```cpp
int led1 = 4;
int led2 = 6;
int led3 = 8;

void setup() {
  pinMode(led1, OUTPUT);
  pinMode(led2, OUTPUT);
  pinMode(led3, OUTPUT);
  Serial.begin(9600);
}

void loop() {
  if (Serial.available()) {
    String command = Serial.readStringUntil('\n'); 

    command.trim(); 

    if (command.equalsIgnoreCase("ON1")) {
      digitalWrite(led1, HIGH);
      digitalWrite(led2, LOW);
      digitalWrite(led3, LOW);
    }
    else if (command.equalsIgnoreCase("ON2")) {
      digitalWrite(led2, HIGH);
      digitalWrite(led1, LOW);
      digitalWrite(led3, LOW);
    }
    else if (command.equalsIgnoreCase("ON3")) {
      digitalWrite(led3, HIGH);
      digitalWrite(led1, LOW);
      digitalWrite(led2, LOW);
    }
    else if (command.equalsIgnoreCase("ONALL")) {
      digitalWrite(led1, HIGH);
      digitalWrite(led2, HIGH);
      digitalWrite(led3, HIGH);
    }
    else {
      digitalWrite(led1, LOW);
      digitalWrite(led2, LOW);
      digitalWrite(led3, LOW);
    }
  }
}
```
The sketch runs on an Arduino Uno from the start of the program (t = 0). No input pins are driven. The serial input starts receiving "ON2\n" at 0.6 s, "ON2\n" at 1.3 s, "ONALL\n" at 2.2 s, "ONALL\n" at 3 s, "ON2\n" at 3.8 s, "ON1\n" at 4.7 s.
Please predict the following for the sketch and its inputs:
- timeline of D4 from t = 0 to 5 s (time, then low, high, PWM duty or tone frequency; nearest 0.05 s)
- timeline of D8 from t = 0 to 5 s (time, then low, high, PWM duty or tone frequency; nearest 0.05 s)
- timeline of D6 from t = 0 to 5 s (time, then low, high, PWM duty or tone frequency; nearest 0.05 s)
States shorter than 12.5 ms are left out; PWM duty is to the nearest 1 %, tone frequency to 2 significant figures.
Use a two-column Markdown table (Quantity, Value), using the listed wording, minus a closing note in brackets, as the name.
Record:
| Quantity | Value |
|---|---|
| timeline of D4 from t = 0 to 5 s | 0 s low; 2.2 s high; 3.8 s low; 4.7 s high |
| timeline of D8 from t = 0 to 5 s | 0 s low; 2.2 s high; 3.8 s low |
| timeline of D6 from t = 0 to 5 s | 0 s low; 0.6 s high; 4.7 s low |
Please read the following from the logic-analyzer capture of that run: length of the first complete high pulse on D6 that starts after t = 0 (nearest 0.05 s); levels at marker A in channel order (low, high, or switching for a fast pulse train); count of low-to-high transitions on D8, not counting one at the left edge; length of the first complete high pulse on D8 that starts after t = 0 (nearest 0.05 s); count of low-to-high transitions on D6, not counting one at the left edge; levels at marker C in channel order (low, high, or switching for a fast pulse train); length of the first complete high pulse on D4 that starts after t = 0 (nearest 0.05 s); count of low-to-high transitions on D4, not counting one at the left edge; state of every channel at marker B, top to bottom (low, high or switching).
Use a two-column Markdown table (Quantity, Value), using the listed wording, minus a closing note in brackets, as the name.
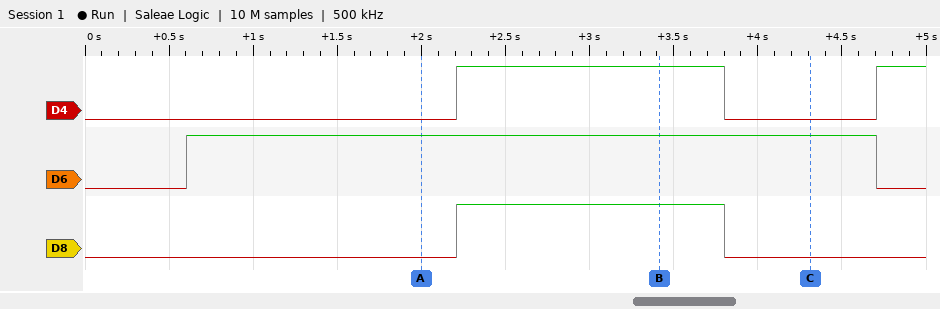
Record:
| Quantity | Value |
|---|---|
| length of the first complete high pulse on D6 that starts after t = 0 | 4.10 s |
| levels at marker A in channel order | D4 low, D6 high, D8 low |
| count of low-to-high transitions on D8, not counting one at the left edge | 1 |
| length of the first complete high pulse on D8 that starts after t = 0 | 1.60 s |
| count of low-to-high transitions on D6, not counting one at the left edge | 1 |
| levels at marker C in channel order | D4 low, D6 high, D8 low |
| length of the first complete high pulse on D4 that starts after t = 0 | 1.60 s |
| count of low-to-high transitions on D4, not counting one at the left edge | 2 |
| state of every channel at marker B, top to bottom | D4 high, D6 high, D8 high |
